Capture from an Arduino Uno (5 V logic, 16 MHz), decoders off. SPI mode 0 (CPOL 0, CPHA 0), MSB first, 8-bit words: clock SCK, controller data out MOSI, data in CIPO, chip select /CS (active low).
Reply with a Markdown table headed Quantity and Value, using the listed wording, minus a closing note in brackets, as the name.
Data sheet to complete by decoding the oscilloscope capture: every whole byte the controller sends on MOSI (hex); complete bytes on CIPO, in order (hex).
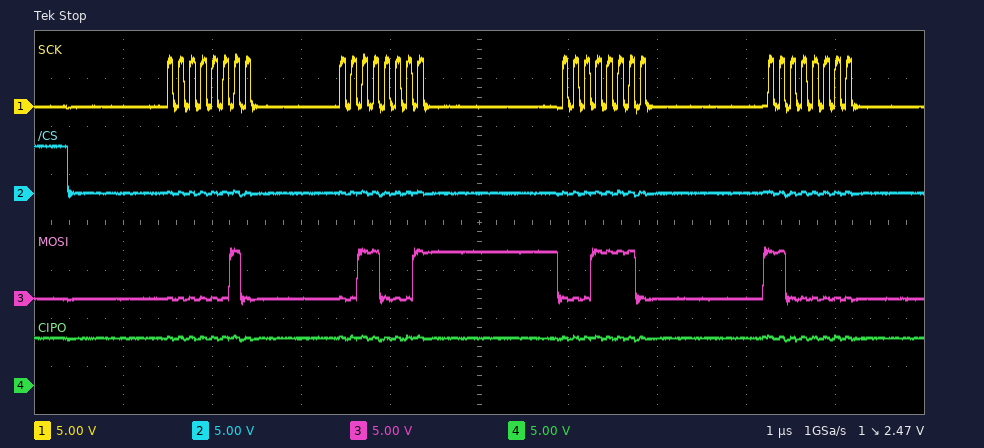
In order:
| Quantity | Value |
|---|---|
| every whole byte the controller sends on MOSI | 02 31 1E C0 |
| complete bytes on CIPO, in order | FF FF FF FF |
